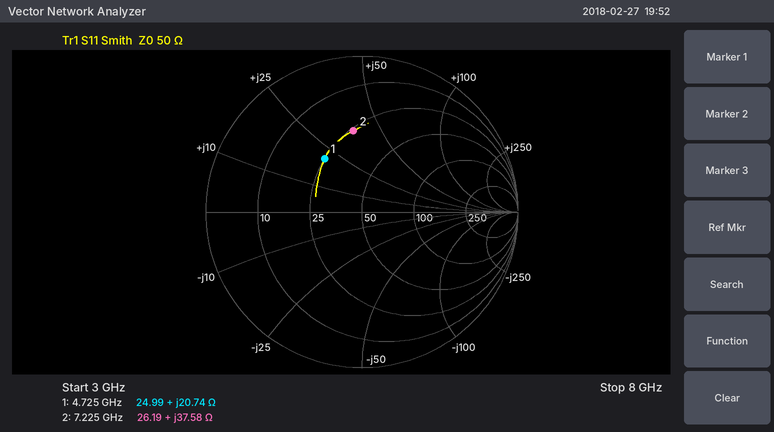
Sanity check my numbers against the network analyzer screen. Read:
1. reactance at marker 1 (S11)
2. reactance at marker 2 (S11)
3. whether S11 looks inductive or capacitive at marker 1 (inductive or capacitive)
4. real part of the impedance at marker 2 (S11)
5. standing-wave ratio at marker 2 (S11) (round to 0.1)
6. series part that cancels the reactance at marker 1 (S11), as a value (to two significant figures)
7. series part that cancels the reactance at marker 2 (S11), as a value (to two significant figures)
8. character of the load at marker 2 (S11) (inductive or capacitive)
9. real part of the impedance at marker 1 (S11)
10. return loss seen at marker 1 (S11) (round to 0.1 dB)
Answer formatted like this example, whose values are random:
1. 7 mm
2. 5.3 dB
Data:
1. +20.74 Ω
2. +37.58 Ω
3. inductive
4. 26.19 Ω
5. 3.2
6. 1.6 pF
7. 590 fF
8. inductive
9. 24.99 Ω
10. 7.6 dB
